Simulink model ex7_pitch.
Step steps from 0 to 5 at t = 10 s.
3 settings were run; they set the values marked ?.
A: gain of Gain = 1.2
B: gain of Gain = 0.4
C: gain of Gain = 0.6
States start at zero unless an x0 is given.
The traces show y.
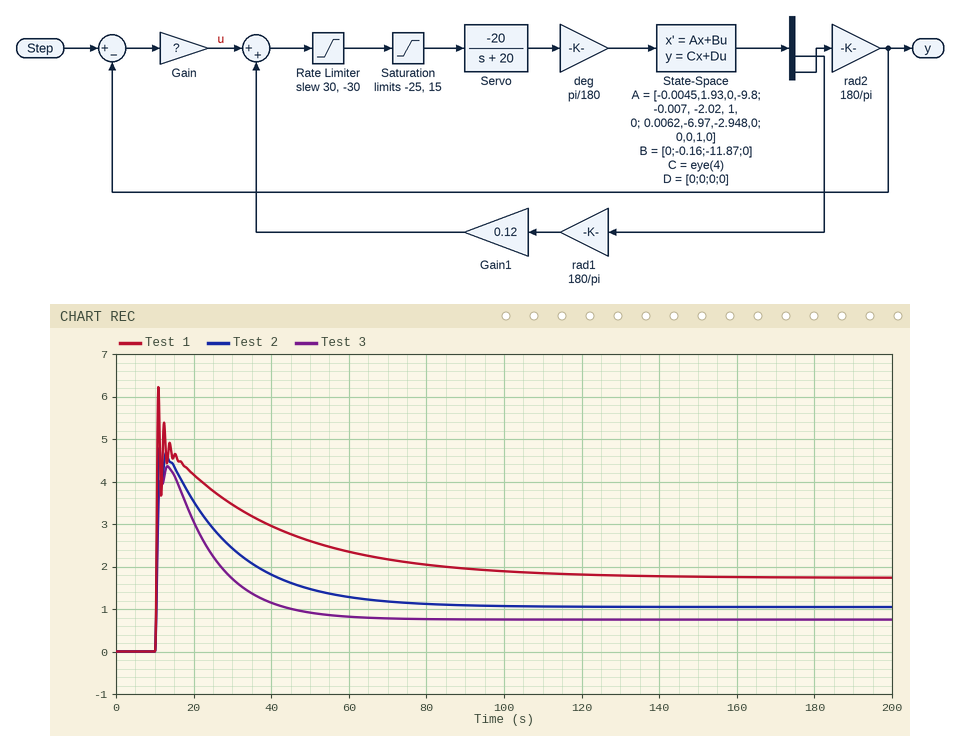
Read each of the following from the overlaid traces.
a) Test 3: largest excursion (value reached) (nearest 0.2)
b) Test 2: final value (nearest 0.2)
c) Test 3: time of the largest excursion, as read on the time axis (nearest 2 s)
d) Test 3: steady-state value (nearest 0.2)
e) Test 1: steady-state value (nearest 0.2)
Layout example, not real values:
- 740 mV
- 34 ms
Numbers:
- 4.4
- 1.0
- 14 s
- 0.8
- 1.8
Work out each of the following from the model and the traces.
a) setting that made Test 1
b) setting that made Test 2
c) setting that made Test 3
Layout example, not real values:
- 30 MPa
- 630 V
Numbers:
- A
- C
- B
